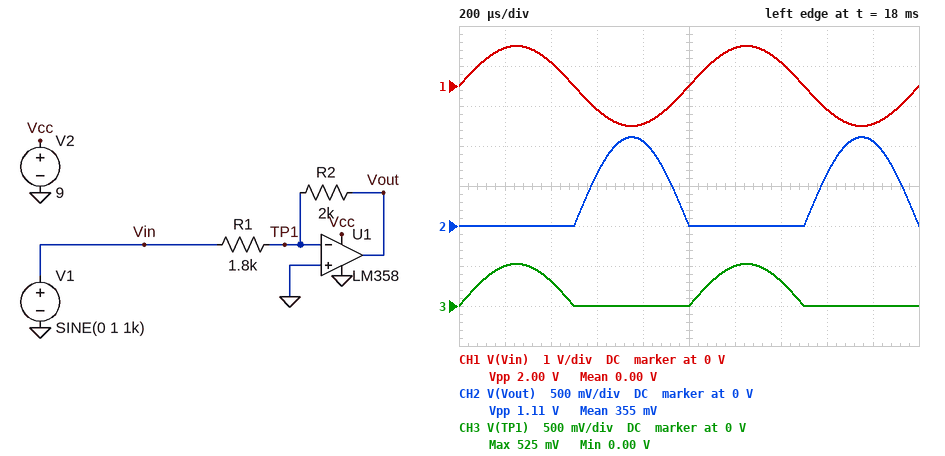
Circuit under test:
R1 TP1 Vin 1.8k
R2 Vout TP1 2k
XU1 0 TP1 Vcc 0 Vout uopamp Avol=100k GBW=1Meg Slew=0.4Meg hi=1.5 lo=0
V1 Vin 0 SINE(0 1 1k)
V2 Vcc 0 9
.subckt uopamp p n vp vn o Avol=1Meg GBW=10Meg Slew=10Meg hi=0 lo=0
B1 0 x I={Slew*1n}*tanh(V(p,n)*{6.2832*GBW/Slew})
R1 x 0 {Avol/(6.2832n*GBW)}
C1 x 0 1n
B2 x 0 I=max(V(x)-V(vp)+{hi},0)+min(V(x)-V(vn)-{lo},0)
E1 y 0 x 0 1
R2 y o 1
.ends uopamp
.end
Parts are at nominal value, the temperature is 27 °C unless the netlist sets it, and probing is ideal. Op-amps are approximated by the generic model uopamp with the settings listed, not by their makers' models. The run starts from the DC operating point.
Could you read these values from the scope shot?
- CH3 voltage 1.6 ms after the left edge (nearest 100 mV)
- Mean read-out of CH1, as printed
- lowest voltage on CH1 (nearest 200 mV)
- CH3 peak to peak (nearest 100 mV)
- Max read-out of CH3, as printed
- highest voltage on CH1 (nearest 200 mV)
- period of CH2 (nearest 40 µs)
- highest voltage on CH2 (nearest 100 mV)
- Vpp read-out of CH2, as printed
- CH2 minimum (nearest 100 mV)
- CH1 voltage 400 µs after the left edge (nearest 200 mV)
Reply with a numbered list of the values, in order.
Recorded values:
1. 0 V
2. 0.00 V
3. -1.0 V
4. 500 mV
5. 525 mV
6. 1.0 V
7. 1.00 ms
8. 1.1 V
9. 1.11 V
10. 0 V
11. 600 mV
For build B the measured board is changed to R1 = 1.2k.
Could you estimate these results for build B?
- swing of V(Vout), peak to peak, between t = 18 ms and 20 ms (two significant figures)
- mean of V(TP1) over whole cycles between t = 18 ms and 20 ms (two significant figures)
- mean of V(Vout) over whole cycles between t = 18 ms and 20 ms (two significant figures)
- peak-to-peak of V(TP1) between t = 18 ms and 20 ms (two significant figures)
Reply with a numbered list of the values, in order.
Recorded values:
1. 1.7 V
2. 200 mV
3. 530 mV
4. 630 mV
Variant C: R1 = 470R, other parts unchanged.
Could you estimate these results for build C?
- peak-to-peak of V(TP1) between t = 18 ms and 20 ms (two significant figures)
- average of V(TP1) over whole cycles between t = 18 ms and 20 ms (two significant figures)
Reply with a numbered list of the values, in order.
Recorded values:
1. 810 mV
2. 260 mV
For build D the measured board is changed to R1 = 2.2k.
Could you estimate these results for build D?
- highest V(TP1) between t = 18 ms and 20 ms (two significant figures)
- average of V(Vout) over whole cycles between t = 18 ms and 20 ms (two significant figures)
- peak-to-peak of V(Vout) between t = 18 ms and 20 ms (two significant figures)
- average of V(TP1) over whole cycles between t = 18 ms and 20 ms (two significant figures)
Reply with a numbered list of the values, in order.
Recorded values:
1. 480 mV
2. 290 mV
3. 910 mV
4. 150 mV
